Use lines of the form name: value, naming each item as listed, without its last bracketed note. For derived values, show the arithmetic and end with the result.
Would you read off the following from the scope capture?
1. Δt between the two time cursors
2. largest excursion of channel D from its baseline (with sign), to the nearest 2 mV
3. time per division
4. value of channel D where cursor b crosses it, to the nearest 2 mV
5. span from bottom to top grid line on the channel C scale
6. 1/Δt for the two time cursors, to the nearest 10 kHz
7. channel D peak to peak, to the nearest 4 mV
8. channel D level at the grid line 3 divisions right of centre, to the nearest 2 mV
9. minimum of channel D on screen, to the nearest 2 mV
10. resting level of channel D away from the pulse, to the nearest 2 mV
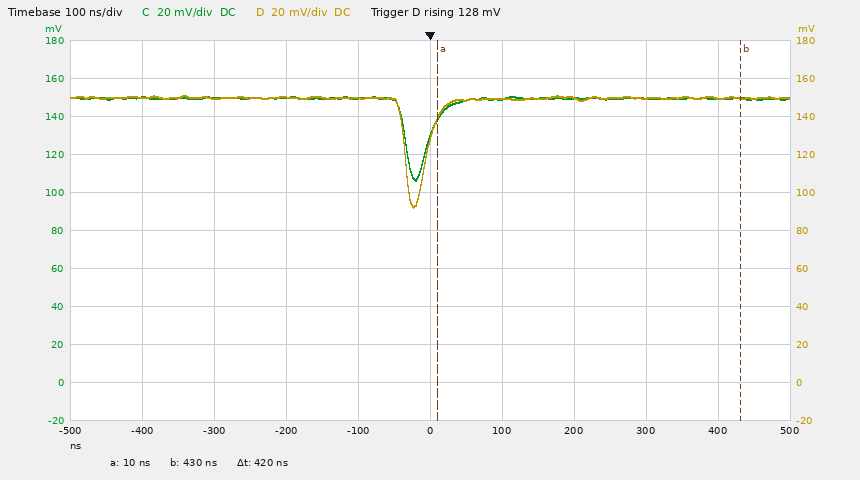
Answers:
Δt between the two time cursors: 420 ns
largest excursion of channel D from its baseline (with sign), to the nearest 2 mV: 92 mV − (150 mV) = -58 mV
time per division: 100 ns
value of channel D where cursor b crosses it, to the nearest 2 mV: 150 mV
span from bottom to top grid line on the channel C scale: 200 mV
1/Δt for the two time cursors, to the nearest 10 kHz: 1 / 420 ns ≈ 2.38 MHz
channel D peak to peak, to the nearest 4 mV: 60 mV
channel D level at the grid line 3 divisions right of centre, to the nearest 2 mV: 150 mV
minimum of channel D on screen, to the nearest 2 mV: 92 mV
resting level of channel D away from the pulse, to the nearest 2 mV: 150 mV
